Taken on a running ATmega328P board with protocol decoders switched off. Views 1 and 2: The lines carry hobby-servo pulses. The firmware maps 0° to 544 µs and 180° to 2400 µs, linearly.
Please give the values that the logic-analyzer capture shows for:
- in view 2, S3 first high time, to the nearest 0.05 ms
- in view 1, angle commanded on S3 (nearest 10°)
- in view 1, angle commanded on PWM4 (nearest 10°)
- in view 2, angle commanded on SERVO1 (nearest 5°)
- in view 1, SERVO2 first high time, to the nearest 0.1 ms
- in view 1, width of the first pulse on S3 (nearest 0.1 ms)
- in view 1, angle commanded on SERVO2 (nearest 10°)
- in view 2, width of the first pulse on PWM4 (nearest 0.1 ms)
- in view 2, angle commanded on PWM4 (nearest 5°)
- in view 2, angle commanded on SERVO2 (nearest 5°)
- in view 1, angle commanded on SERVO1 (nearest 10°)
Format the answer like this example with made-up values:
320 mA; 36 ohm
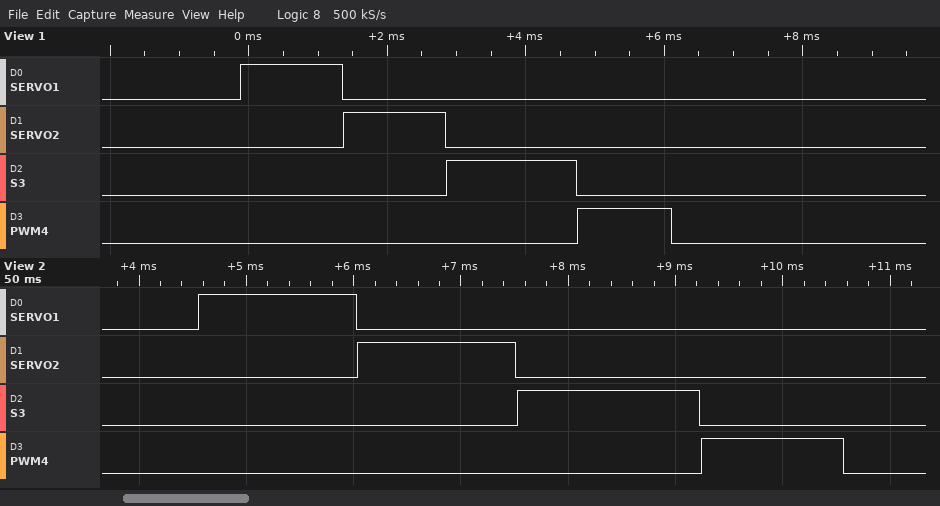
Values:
1.70 ms; 130°; 80°; 90°; 1.5 ms; 1.9 ms; 90°; 1.3 ms; 75°; 90°; 90°
